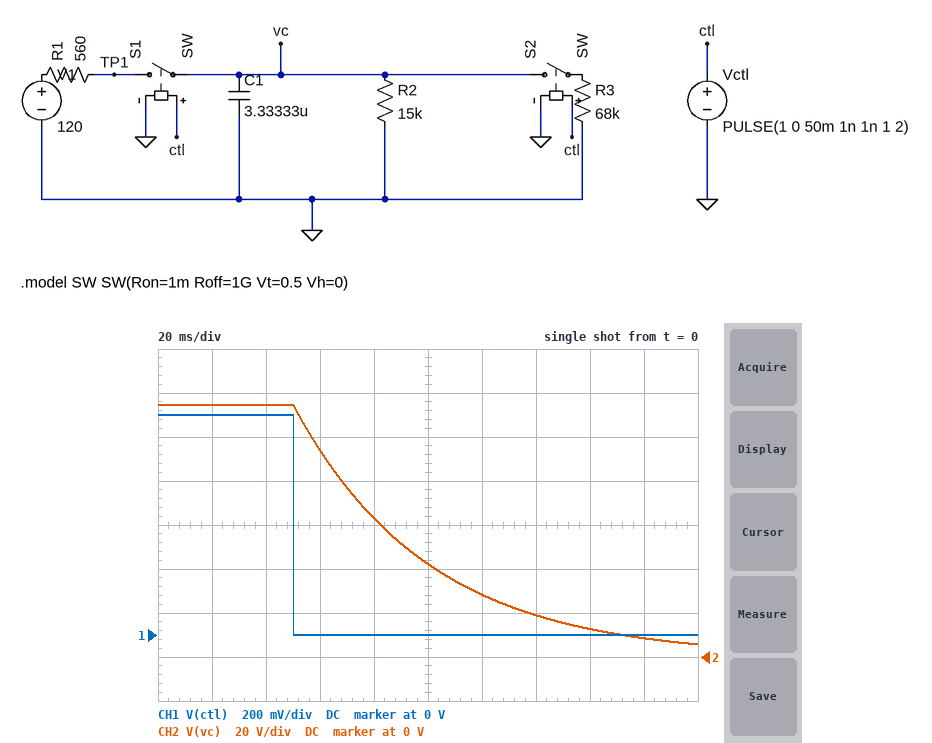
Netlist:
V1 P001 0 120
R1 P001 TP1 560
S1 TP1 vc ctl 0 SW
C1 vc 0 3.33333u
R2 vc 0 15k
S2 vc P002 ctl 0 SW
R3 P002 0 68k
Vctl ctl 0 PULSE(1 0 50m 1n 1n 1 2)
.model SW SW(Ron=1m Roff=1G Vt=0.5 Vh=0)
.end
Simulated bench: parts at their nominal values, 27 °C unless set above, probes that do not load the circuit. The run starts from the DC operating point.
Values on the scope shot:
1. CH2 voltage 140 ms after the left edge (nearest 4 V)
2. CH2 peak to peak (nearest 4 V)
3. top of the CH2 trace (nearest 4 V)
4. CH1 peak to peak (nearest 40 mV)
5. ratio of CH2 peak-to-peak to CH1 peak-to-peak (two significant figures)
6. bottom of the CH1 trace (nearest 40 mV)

20 V
108 V
116 V
1.00 V
110
0 V
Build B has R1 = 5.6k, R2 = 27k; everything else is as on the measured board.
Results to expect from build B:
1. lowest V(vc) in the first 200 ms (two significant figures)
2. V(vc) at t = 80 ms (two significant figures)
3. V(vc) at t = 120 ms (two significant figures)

18 V
67 V
43 V
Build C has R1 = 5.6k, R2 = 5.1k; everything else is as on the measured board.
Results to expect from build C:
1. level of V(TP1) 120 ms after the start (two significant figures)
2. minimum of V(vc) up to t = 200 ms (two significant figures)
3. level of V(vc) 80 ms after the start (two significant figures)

120 V
8.7 mV
9.4 V
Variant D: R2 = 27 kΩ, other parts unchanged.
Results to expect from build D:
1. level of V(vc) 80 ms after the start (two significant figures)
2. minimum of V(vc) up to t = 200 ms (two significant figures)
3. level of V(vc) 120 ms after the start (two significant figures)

84 V
22 V
54 V
